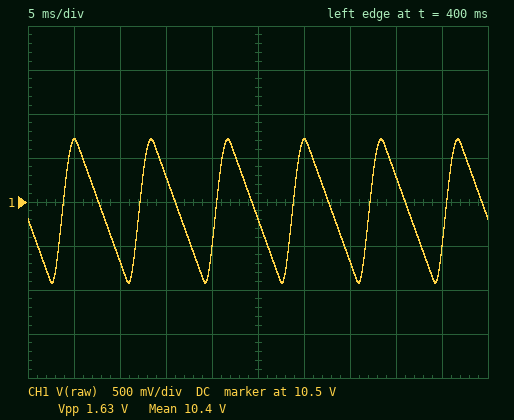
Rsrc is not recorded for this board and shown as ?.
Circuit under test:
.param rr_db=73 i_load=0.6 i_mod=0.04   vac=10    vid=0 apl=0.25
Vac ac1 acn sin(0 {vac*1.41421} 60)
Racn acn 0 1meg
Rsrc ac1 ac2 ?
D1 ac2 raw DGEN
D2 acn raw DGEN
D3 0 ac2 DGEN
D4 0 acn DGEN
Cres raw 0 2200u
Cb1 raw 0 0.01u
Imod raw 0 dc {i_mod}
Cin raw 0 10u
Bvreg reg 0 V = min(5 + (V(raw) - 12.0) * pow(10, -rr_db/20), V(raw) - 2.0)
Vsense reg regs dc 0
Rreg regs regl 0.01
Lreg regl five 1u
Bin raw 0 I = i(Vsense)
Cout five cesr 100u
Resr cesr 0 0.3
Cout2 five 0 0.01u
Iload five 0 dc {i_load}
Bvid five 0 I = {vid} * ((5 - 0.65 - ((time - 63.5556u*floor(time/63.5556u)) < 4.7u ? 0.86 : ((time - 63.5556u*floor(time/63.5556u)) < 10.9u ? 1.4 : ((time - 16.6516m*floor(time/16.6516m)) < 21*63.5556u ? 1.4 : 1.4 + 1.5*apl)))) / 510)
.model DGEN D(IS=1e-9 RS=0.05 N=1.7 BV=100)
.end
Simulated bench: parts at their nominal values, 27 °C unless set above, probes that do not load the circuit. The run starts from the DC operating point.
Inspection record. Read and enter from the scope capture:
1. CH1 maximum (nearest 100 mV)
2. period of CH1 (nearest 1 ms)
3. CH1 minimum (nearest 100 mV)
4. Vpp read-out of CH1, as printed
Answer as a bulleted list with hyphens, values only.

- 11.2 V
- 8 ms
- 9.6 V
- 1.63 V
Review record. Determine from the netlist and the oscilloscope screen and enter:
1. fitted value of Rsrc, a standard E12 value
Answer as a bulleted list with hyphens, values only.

- 0.47 Ω
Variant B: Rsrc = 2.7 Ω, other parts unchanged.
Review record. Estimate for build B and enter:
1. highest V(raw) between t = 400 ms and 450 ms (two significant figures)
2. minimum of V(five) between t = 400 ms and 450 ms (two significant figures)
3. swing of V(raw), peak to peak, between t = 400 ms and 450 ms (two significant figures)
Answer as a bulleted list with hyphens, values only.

- 7.9 V
- 4.7 V
- 1.2 V
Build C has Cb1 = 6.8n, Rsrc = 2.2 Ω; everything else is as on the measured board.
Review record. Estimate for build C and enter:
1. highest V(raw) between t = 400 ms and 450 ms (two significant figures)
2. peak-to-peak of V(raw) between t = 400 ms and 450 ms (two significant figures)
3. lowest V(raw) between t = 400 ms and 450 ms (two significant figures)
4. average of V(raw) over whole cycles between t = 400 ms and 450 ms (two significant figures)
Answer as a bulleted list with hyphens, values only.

- 8.6 V
- 1.3 V
- 7.3 V
- 7.9 V
